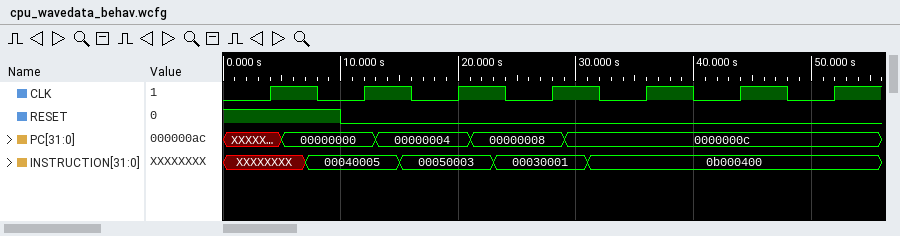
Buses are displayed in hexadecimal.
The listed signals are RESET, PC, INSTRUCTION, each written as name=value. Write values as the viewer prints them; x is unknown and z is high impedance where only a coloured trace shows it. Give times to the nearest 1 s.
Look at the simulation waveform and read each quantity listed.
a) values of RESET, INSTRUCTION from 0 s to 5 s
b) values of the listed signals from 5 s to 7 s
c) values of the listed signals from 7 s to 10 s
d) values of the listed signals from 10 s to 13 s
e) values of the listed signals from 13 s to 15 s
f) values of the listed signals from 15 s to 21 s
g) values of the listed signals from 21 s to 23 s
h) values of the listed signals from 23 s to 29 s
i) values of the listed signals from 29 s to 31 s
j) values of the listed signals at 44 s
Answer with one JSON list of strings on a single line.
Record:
["RESET=1, INSTRUCTION=XXXXXXXX", "RESET=1, PC=00000000, INSTRUCTION=XXXXXXXX", "RESET=1, PC=00000000, INSTRUCTION=00040005", "RESET=0, PC=00000000, INSTRUCTION=00040005", "RESET=0, PC=00000004, INSTRUCTION=00040005", "RESET=0, PC=00000004, INSTRUCTION=00050003", "RESET=0, PC=00000008, INSTRUCTION=00050003", "RESET=0, PC=00000008, INSTRUCTION=00030001", "RESET=0, PC=0000000c, INSTRUCTION=00030001", "RESET=0, PC=0000000c, INSTRUCTION=0b000400"]
